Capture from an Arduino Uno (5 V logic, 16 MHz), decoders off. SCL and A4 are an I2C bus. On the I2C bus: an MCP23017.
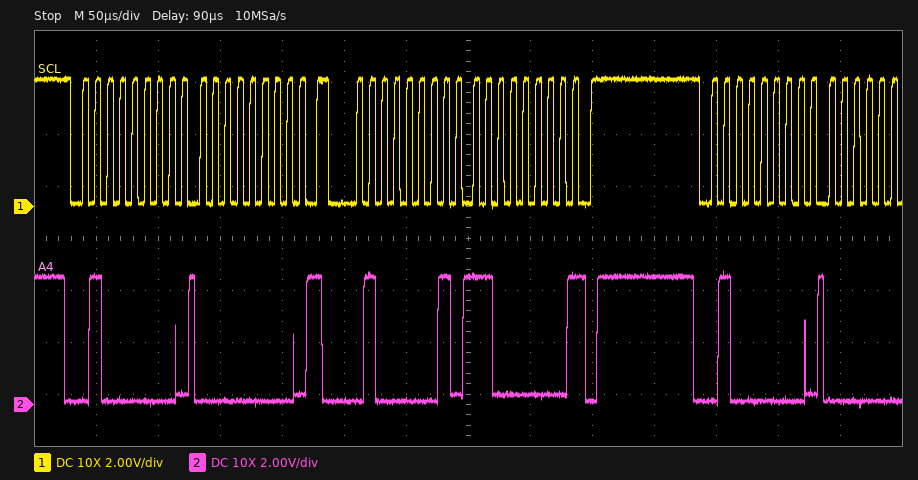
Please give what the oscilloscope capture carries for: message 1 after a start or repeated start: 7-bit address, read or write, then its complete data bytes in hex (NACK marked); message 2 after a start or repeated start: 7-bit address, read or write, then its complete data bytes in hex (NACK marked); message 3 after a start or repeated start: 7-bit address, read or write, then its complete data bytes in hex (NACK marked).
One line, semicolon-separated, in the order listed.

0x20 write: 00; 0x20 read: C0 NACK; 0x20 write
